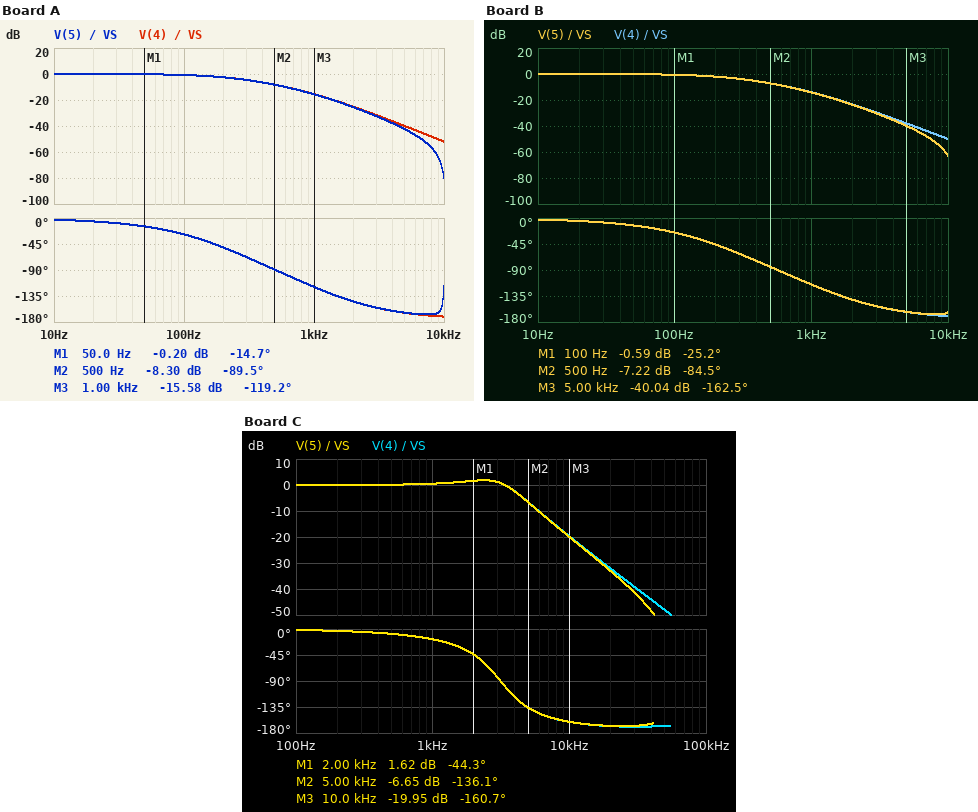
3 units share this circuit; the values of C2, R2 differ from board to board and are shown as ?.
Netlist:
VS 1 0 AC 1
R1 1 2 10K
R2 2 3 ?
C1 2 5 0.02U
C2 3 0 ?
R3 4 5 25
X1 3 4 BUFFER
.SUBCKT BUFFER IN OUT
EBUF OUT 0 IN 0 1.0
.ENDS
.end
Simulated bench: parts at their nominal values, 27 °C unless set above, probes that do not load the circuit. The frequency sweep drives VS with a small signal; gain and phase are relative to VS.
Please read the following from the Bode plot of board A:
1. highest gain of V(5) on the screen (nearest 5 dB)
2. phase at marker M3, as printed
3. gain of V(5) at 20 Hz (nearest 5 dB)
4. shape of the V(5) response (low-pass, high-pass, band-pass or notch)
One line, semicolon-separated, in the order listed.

0 dB; -119.2 deg; 0 dB; low-pass
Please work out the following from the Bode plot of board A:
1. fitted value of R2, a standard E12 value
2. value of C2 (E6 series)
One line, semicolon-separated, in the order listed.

15 kΩ; 33 nF
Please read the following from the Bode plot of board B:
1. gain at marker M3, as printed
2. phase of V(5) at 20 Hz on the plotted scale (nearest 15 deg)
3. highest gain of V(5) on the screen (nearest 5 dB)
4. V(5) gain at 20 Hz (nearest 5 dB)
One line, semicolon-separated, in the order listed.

-40.04 dB; 0 deg; 0 dB; 0 dB
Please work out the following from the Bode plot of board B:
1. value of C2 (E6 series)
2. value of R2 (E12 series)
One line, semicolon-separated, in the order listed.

33 nF; 12 kΩ
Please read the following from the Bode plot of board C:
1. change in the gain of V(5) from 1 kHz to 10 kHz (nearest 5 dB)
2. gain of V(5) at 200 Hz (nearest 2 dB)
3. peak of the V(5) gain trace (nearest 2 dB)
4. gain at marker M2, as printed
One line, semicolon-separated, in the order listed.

-20 dB; 0 dB; 2 dB; -6.65 dB
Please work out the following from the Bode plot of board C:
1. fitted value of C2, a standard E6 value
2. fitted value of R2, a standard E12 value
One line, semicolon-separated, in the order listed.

3.3 nF; 3.9 kΩ
